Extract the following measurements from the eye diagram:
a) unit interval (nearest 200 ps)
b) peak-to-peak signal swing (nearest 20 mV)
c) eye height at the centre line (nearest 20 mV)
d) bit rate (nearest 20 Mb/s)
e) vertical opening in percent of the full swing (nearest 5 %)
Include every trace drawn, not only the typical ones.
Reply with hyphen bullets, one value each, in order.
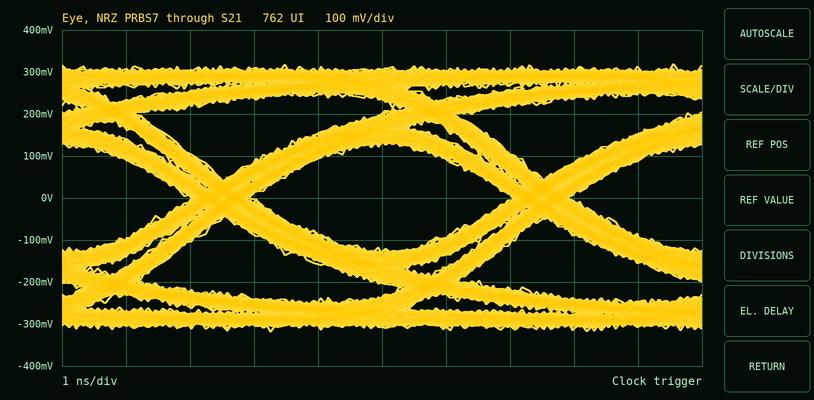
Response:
- 5.0 ns
- 640 mV
- 260 mV
- 200 Mb/s
- 40 %
